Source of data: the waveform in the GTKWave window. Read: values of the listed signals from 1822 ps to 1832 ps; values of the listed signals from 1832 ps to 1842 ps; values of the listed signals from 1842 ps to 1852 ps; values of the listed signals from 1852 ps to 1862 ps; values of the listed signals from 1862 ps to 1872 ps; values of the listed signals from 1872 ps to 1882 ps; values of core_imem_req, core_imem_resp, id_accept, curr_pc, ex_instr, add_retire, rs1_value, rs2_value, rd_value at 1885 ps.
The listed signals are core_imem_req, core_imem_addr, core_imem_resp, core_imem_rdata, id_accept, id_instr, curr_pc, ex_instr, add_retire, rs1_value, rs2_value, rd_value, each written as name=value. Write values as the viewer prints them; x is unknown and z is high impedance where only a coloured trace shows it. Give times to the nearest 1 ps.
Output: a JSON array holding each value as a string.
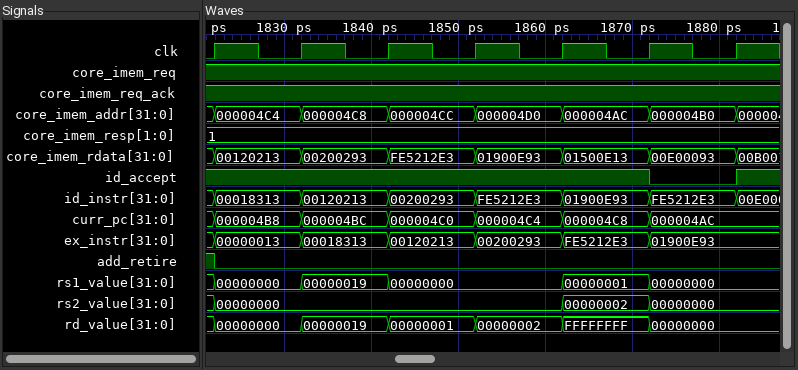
["core_imem_req=1, core_imem_addr=000004C4, core_imem_resp=1, core_imem_rdata=00120213, id_accept=1, id_instr=00018313, curr_pc=000004B8, ex_instr=00000013, add_retire=0, rs1_value=00000000, rs2_value=00000000, rd_value=00000000", "core_imem_req=1, core_imem_addr=000004C8, core_imem_resp=1, core_imem_rdata=00200293, id_accept=1, id_instr=00120213, curr_pc=000004BC, ex_instr=00018313, add_retire=0, rs1_value=00000019, rs2_value=00000000, rd_value=00000019", "core_imem_req=1, core_imem_addr=000004CC, core_imem_resp=1, core_imem_rdata=FE5212E3, id_accept=1, id_instr=00200293, curr_pc=000004C0, ex_instr=00120213, add_retire=0, rs1_value=00000000, rs2_value=00000000, rd_value=00000001", "core_imem_req=1, core_imem_addr=000004D0, core_imem_resp=1, core_imem_rdata=01900E93, id_accept=1, id_instr=FE5212E3, curr_pc=000004C4, ex_instr=00200293, add_retire=0, rs1_value=00000000, rs2_value=00000000, rd_value=00000002", "core_imem_req=1, core_imem_addr=000004AC, core_imem_resp=1, core_imem_rdata=01500E13, id_accept=1, id_instr=01900E93, curr_pc=000004C8, ex_instr=FE5212E3, add_retire=0, rs1_value=00000001, rs2_value=00000002, rd_value=FFFFFFFF", "core_imem_req=1, core_imem_addr=000004B0, core_imem_resp=1, core_imem_rdata=00E00093, id_accept=0, id_instr=FE5212E3, curr_pc=000004AC, ex_instr=01900E93, add_retire=0, rs1_value=00000000, rs2_value=00000000, rd_value=00000000", "core_imem_req=1, core_imem_resp=1, id_accept=1, curr_pc=000004AC, ex_instr=01900E93, add_retire=0, rs1_value=00000000, rs2_value=00000000, rd_value=00000000"]
